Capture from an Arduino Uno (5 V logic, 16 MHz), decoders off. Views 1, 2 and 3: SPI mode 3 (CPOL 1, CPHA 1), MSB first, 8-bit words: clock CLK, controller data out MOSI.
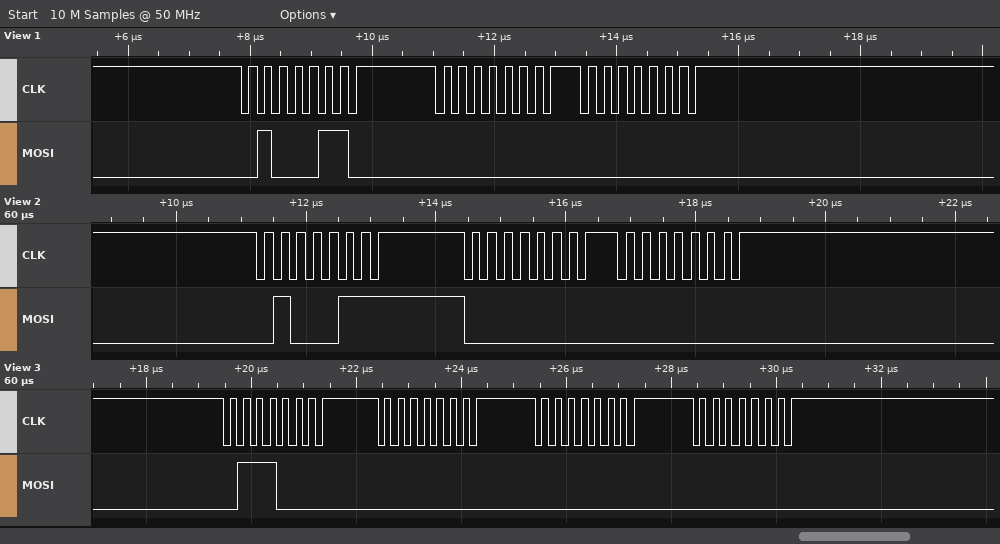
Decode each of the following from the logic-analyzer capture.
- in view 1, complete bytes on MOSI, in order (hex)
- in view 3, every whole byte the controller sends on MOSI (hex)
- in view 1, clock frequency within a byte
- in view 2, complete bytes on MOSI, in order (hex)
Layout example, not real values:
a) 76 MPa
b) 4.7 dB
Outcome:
a) 46 00 00
b) 0x70 0x00 0x00 0x00
c) 4 MHz
d) 47 00 00
